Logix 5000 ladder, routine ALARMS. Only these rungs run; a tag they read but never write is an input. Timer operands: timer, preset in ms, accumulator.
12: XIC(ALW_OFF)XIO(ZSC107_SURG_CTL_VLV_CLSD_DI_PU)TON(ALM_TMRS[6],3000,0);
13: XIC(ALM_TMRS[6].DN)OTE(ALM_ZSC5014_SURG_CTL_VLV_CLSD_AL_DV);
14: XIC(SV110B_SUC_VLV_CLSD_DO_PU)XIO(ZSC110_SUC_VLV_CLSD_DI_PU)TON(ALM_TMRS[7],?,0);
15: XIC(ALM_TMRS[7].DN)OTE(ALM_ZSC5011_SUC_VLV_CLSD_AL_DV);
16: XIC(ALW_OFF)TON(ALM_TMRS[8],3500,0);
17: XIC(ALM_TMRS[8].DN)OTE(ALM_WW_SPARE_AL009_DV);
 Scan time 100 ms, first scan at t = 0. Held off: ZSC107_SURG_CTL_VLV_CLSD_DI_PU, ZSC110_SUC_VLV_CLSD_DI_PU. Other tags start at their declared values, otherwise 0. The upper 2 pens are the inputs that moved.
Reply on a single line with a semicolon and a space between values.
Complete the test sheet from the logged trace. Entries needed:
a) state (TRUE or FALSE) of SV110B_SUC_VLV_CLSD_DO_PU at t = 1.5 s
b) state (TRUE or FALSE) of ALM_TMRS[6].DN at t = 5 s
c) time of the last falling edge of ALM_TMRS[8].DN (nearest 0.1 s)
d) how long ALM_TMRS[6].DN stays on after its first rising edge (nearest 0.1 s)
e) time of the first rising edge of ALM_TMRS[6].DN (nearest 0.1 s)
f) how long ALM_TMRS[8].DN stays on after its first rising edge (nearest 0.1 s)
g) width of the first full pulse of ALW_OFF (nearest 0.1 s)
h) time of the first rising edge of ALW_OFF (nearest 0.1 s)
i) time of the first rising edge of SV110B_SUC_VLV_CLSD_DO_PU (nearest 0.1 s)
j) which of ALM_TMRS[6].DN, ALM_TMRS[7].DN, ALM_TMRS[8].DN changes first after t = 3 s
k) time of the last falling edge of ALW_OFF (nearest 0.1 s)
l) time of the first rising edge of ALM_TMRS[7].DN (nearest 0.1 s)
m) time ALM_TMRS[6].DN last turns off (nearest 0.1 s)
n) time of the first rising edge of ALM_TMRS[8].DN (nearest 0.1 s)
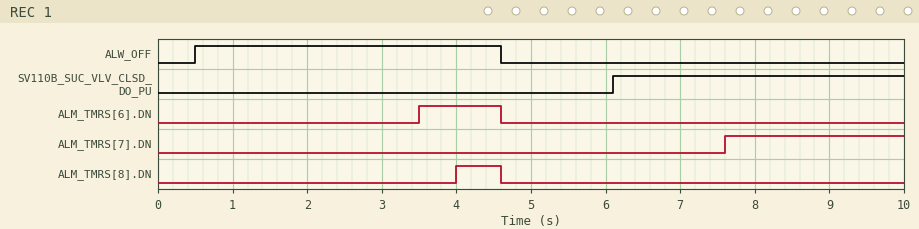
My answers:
FALSE; FALSE; 4.6 s; 1.1 s; 3.5 s; 0.6 s; 4.1 s; 0.5 s; 6.1 s; ALM_TMRS[6].DN; 4.6 s; 7.6 s; 4.6 s; 4.0 s
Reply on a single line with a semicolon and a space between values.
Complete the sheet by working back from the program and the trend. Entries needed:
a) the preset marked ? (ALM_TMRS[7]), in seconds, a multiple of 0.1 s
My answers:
1.5 s
